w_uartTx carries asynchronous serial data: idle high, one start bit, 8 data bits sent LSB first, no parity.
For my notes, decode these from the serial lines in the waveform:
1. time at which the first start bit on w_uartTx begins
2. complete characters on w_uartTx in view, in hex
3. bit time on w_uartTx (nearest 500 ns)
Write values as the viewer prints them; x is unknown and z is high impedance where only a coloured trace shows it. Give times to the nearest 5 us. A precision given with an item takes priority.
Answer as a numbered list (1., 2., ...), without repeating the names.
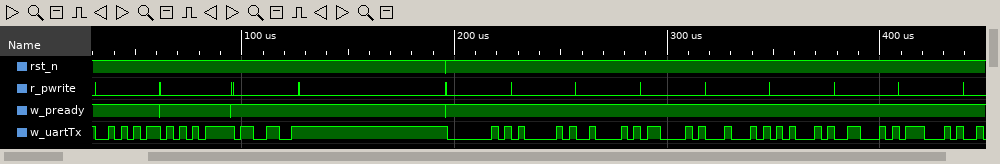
1. 30 us
2. AA, D5, 33, 40, 41, 42, 43, 44, 45, 46, 47
3. 3000 ns
